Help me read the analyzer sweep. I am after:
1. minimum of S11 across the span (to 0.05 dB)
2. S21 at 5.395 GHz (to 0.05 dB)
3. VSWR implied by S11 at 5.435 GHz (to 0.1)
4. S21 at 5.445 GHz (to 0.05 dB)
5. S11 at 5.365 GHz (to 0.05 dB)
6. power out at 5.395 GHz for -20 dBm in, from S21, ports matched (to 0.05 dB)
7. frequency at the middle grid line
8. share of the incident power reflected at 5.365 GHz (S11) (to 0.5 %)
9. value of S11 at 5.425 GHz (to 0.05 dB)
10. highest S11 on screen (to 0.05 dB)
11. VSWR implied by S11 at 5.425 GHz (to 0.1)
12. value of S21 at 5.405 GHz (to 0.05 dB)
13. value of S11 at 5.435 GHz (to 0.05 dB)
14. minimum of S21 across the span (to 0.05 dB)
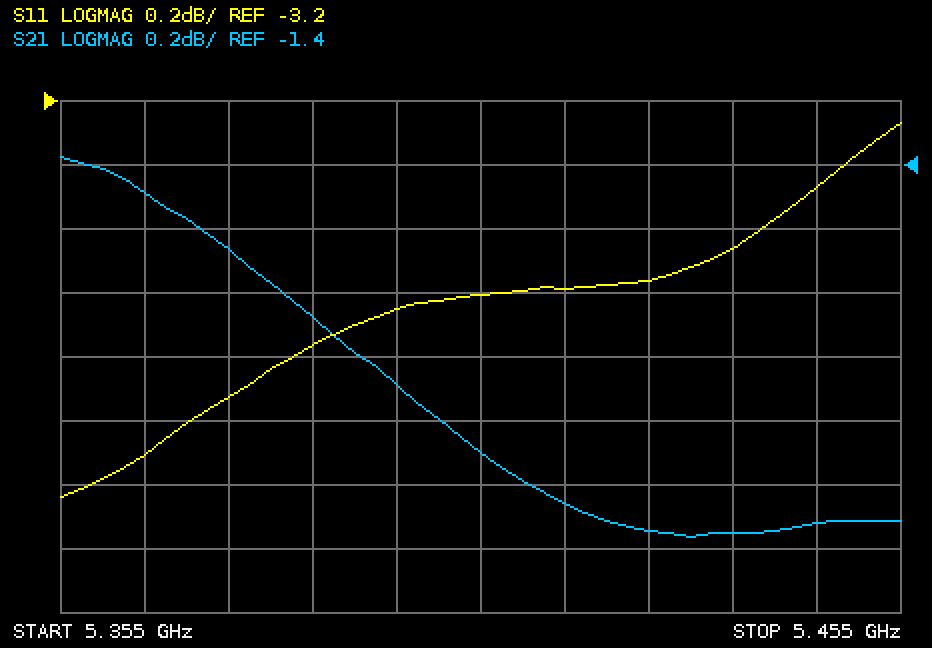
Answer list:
-4.45 dB
-2.10 dB
4.8
-2.50 dB
-4.30 dB
-22.10 dBm
5.405 GHz
37.0 %
-3.75 dB
-3.25 dB
4.7
-2.30 dB
-3.65 dB
-2.55 dB
